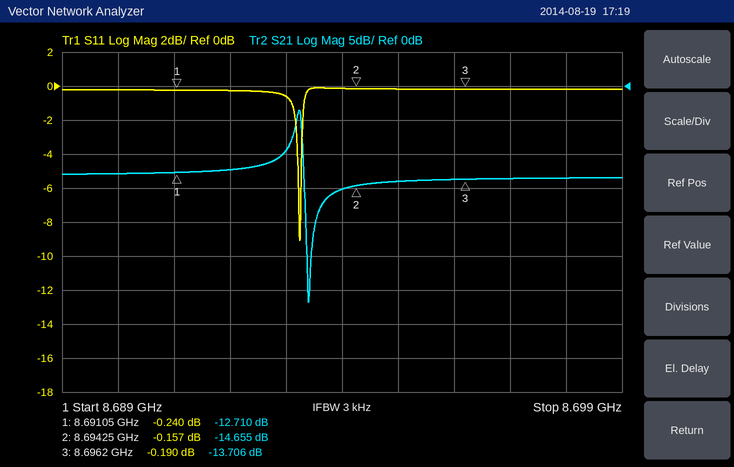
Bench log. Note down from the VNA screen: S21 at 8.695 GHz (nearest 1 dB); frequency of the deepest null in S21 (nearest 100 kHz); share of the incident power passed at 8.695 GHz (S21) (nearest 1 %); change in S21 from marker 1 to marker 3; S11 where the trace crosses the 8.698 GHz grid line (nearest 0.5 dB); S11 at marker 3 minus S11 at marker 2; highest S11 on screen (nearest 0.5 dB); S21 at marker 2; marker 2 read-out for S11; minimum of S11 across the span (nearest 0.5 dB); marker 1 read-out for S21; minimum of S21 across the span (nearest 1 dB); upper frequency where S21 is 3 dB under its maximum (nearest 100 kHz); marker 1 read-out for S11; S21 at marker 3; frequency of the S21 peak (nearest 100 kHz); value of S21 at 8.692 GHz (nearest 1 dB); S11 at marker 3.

-14 dB
8.6934 GHz
4 %
-0.996 dB
0.0 dB
-0.033 dB
0.0 dB
-14.655 dB
-0.157 dB
-9.0 dB
-12.710 dB
-32 dB
8.6933 GHz
-0.240 dB
-13.706 dB
8.6932 GHz
-12 dB
-0.190 dB
